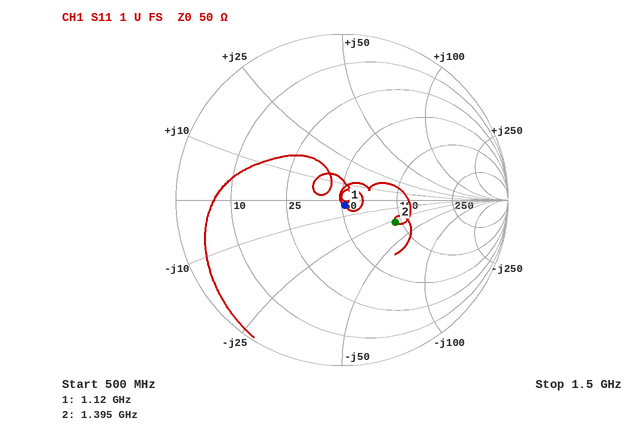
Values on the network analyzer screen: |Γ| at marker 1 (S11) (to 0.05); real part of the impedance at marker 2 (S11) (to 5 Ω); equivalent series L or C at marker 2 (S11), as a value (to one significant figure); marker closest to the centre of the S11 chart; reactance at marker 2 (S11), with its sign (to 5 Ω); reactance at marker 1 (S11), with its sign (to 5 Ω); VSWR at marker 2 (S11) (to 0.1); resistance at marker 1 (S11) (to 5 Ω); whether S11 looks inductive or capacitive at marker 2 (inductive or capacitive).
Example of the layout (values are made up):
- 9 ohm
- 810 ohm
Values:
- 0.05
- 90 Ω
- 4 pF
- marker 1
- -30 Ω
- -5 Ω
- 2.1
- 50 Ω
- capacitive
